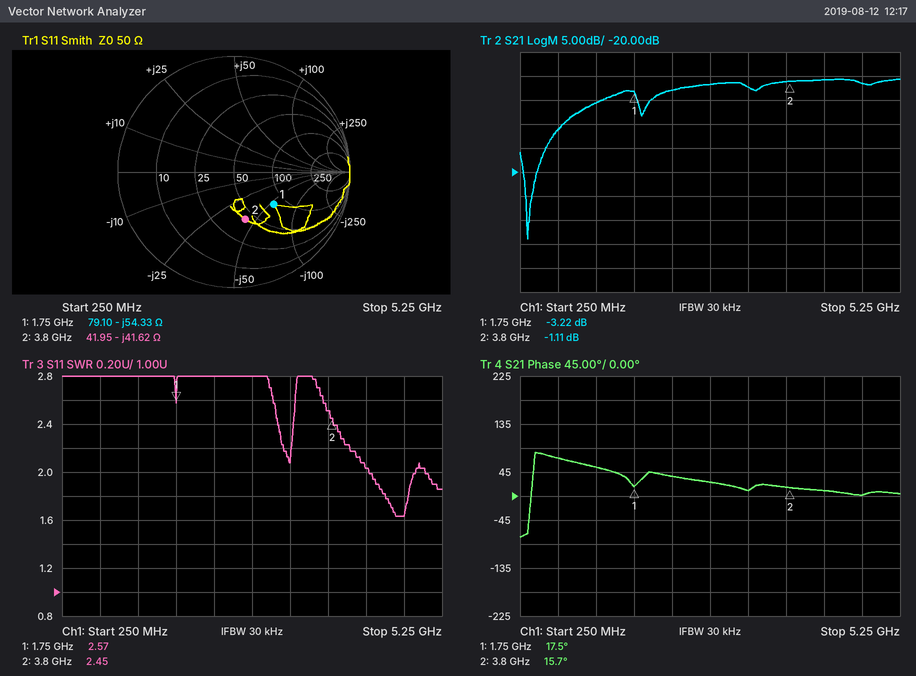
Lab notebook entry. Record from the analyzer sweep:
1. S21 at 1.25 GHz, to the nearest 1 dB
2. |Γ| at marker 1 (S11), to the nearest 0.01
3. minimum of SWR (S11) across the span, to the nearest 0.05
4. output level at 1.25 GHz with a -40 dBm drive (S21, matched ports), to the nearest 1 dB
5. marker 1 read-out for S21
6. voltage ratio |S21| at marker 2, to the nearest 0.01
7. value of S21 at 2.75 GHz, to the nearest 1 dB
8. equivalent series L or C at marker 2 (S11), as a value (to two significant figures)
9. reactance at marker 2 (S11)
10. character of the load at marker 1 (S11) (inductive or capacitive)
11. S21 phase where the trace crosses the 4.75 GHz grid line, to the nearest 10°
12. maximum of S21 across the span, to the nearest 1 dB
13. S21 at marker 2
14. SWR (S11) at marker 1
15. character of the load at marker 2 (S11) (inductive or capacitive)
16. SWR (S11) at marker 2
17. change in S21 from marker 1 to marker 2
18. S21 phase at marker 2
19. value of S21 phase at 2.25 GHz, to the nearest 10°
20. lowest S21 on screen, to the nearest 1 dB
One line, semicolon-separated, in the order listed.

-6 dB; 0.44; 1.65; -46 dBm; -3.22 dB; 0.88; -2 dB; 1.0 pF; -41.62 Ω; capacitive; 0°; -1 dB; -1.11 dB; 2.57; capacitive; 2.45; 2.11 dB; 15.7°; 40°; -34 dB
